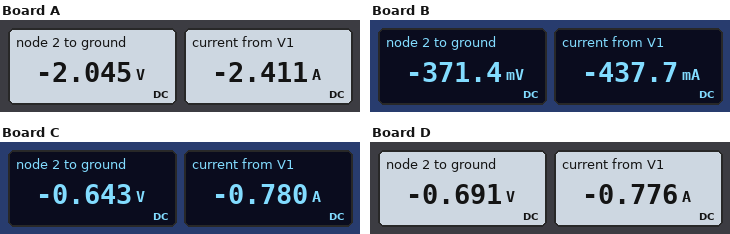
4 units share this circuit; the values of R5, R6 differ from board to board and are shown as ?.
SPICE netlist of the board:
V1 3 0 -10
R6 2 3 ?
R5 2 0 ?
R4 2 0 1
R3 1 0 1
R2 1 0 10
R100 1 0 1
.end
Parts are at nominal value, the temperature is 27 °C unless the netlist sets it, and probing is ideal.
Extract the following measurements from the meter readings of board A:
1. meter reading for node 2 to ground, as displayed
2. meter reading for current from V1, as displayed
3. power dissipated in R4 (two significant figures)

-2.045 V
-2.411 A
4.2 W
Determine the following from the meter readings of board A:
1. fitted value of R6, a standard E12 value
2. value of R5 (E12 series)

3.3 Ω
5.6 Ω
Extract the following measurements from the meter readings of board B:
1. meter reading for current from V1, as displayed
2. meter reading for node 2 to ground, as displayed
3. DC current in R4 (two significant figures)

-437.7 mA
-371.4 mV
370 mA
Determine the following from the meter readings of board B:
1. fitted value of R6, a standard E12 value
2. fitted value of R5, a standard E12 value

22 Ω
5.6 Ω
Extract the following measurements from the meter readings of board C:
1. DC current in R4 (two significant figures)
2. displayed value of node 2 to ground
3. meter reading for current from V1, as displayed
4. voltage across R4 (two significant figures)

640 mA
-0.643 V
-0.780 A
640 mV
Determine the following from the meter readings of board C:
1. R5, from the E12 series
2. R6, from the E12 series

4.7 Ω
12 Ω
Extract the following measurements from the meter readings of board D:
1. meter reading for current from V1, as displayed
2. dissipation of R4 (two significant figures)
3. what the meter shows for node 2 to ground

-0.776 A
480 mW
-0.691 V
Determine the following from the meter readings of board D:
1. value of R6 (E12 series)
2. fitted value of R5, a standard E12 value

12 Ω
8.2 Ω
